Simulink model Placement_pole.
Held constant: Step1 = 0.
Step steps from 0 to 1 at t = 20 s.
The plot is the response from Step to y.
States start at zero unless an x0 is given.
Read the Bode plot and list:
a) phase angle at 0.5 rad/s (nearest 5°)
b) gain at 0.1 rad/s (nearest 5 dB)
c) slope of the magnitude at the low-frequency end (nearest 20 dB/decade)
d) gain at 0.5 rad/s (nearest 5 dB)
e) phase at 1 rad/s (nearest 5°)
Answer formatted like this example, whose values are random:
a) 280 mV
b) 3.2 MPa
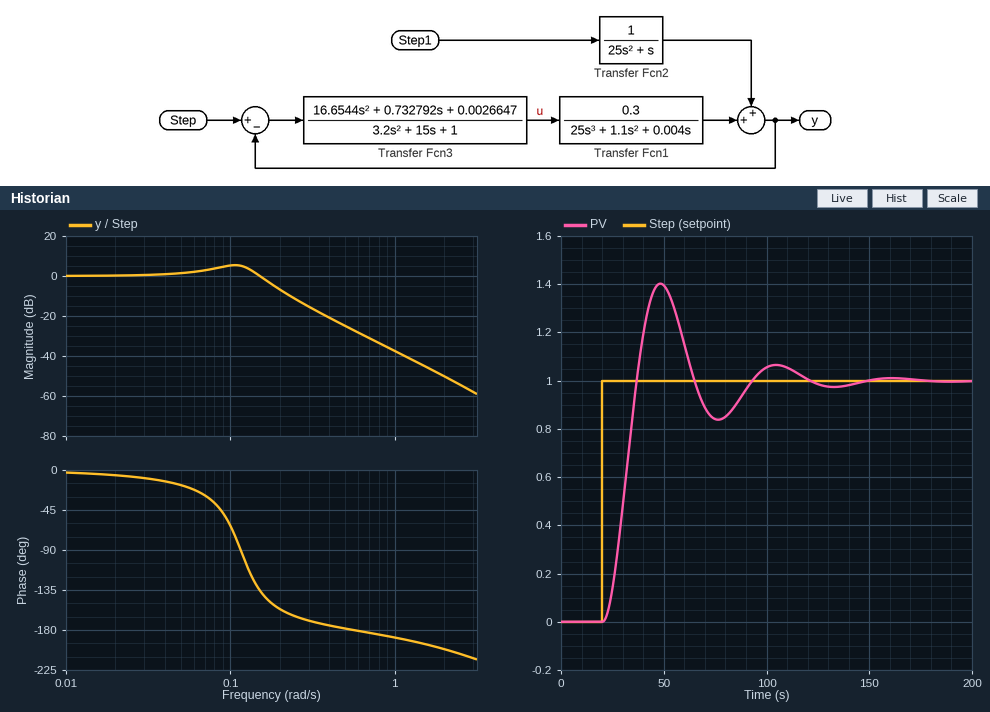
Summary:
a) -180°
b) 5 dB
c) 0 dB/decade
d) -25 dB
e) -190°
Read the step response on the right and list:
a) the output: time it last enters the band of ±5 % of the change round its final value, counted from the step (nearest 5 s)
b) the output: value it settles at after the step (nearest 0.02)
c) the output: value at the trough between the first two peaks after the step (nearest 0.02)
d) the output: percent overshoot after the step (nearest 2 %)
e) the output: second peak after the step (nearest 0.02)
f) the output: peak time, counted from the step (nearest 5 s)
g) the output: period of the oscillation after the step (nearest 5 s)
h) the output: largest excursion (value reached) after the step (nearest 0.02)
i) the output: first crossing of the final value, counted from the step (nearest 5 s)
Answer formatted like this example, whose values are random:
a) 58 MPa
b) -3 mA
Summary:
a) 90 s
b) 1.00
c) 0.84
d) 40 %
e) 1.06
f) 30 s
g) 55 s
h) 1.40
i) 15 s
